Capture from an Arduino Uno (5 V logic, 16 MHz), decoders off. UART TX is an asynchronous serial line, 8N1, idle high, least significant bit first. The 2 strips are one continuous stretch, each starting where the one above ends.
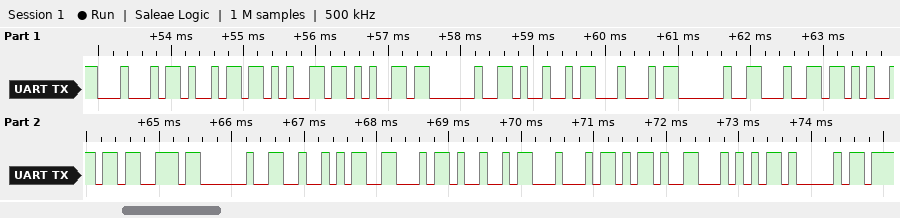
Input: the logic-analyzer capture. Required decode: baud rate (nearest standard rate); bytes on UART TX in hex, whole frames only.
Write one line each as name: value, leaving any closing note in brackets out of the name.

baud rate: 9600 baud
bytes on UART TX in hex, whole frames only: 0x44 0x69 0x65 0x65 0x20 0x49 0x44 0x20 0x64 0x65 0x73 0x20 0x52 0x46 0x49 0x44 0x2D 0x54 0x41
